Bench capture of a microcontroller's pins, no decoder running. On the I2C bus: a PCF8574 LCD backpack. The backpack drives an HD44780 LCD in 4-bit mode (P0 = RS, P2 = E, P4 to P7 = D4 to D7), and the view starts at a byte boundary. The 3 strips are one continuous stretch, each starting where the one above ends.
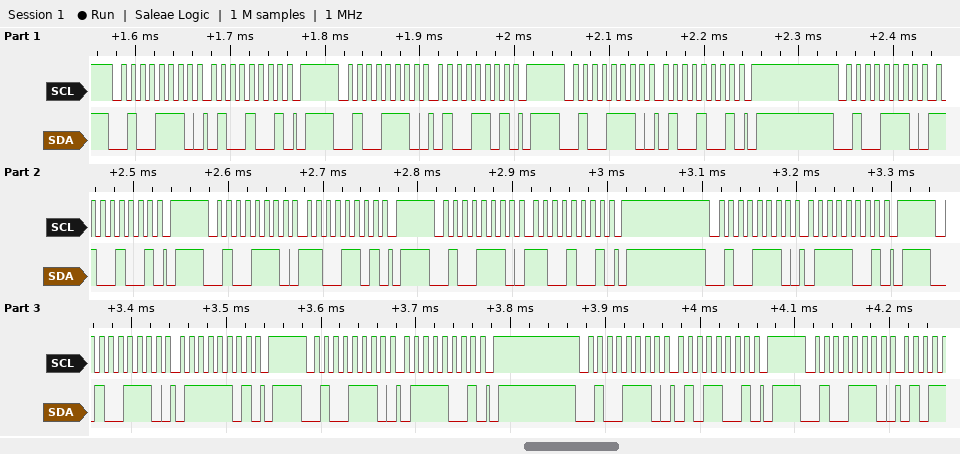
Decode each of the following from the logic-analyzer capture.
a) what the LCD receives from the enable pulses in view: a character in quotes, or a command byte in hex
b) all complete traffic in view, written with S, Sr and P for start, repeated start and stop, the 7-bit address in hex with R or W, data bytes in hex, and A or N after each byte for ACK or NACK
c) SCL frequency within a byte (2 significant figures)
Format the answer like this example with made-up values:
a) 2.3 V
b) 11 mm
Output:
a) 'L'
b) S 27W A 49 A P S 27W A 4D A P S 27W A 49 A P S 27W A C9 A P S 27W A CD A P S 27W A C9 A P S 27W A 79 A P S 27W A 7D A P S 27W A 79 A P S 27W A 59 A P S 27W A
c) 100 kHz
